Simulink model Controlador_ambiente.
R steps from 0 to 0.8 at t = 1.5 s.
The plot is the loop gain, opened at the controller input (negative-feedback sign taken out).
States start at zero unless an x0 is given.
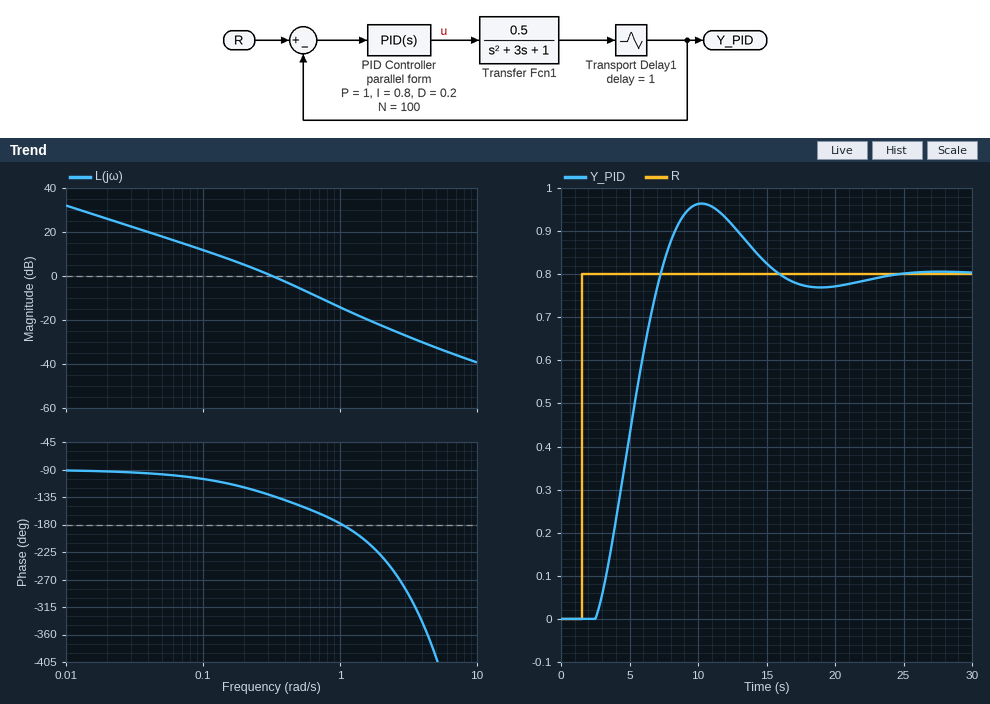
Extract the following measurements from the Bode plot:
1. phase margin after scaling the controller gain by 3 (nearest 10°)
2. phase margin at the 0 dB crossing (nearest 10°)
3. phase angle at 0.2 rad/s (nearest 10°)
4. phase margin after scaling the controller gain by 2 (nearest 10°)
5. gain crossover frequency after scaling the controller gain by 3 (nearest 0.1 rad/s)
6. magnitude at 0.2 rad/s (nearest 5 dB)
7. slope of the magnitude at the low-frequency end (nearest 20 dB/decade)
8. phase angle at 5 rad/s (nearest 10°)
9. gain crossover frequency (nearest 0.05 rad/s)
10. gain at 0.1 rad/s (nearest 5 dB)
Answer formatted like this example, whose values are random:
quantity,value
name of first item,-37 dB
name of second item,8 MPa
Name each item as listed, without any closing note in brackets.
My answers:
quantity,value
phase margin after scaling the controller gain by 3,20°
phase margin at the 0 dB crossing,50°
phase angle at 0.2 rad/s,-120°
phase margin after scaling the controller gain by 2,30°
gain crossover frequency after scaling the controller gain by 3,0.7 rad/s
magnitude at 0.2 rad/s,5 dB
slope of the magnitude at the low-frequency end,-20 dB/decade
phase angle at 5 rad/s,-400°
gain crossover frequency,0.30 rad/s
gain at 0.1 rad/s,10 dB
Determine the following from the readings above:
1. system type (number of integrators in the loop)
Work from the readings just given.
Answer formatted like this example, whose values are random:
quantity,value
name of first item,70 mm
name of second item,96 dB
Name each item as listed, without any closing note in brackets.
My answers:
quantity,value
system type,1
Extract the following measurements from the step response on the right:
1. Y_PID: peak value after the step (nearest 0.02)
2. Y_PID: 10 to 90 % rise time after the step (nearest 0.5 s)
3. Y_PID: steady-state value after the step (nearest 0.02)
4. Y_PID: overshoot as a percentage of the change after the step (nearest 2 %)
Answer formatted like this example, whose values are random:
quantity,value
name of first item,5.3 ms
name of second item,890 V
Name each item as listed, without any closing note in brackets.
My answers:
quantity,value
Y_PID: peak value after the step,0.96
Y_PID: 10 to 90 % rise time after the step,3.5 s
Y_PID: steady-state value after the step,0.80
Y_PID: overshoot as a percentage of the change after the step,20 %
